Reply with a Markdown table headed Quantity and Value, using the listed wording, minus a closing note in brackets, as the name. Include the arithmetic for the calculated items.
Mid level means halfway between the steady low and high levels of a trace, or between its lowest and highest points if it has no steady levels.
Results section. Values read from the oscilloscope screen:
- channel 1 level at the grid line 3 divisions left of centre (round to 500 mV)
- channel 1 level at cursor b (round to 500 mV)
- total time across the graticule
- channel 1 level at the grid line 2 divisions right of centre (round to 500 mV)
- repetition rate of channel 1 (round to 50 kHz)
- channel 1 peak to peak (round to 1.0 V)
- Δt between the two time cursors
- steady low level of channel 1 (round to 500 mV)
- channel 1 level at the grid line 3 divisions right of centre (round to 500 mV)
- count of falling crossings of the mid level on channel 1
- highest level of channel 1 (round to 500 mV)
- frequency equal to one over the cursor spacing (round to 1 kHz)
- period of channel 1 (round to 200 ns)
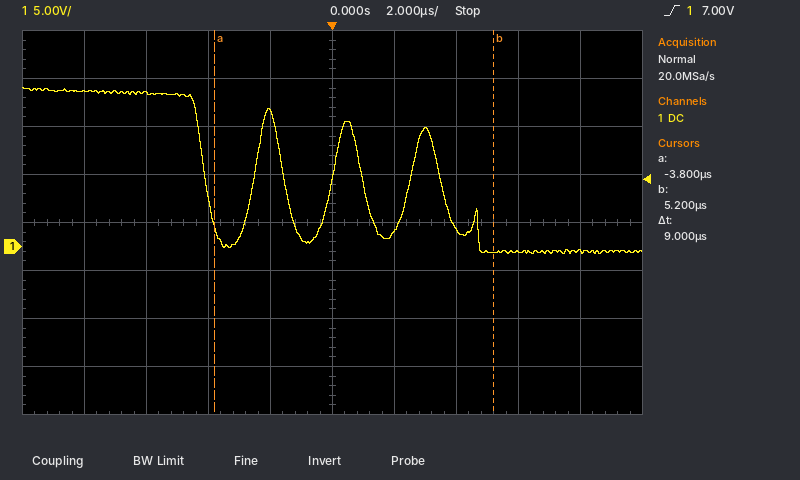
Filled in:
| Quantity | Value |
|---|---|
| channel 1 level at the grid line 3 divisions left of centre | 16.0 V |
| channel 1 level at cursor b | -500 mV |
| total time across the graticule | 20 µs |
| channel 1 level at the grid line 2 divisions right of centre | 2.0 V |
| repetition rate of channel 1 | 1 / 2.6 µs ≈ 385 kHz, so 400 kHz to the nearest 50 kHz |
| channel 1 peak to peak | 17.0 V |
| Δt between the two time cursors | 9 µs |
| steady low level of channel 1 | -500 mV |
| channel 1 level at the grid line 3 divisions right of centre | -500 mV |
| count of falling crossings of the mid level on channel 1 | 4 |
| highest level of channel 1 | 16.5 V |
| frequency equal to one over the cursor spacing | 1 / 9 µs ≈ 111 kHz |
| period of channel 1 | 2.6 µs |
